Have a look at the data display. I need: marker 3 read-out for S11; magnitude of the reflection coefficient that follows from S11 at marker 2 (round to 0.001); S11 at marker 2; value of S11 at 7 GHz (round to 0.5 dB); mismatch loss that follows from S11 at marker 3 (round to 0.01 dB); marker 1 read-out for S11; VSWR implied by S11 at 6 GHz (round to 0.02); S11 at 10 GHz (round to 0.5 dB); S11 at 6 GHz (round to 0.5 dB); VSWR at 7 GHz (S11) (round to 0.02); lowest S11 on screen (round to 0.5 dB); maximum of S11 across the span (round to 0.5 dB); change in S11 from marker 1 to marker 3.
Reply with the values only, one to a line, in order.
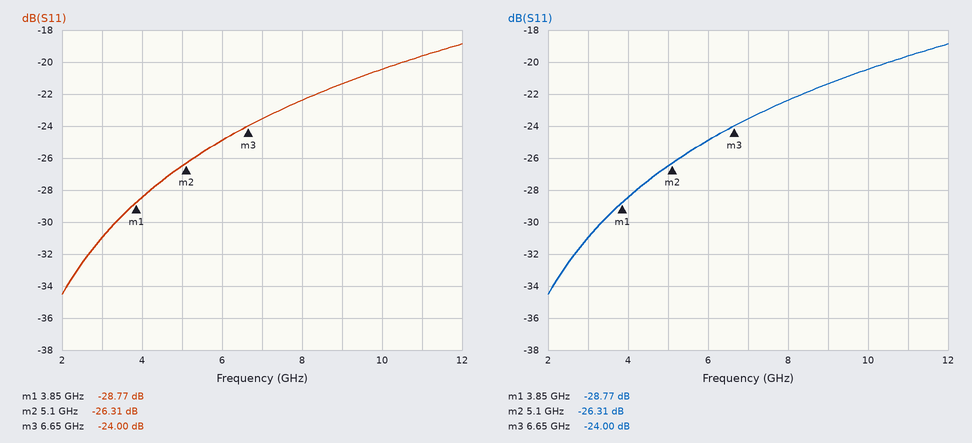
-24.00 dB
0.048
-26.31 dB
-23.5 dB
0.02 dB
-28.77 dB
1.12
-20.5 dB
-25.0 dB
1.14
-34.5 dB
-19.0 dB
4.77 dB
